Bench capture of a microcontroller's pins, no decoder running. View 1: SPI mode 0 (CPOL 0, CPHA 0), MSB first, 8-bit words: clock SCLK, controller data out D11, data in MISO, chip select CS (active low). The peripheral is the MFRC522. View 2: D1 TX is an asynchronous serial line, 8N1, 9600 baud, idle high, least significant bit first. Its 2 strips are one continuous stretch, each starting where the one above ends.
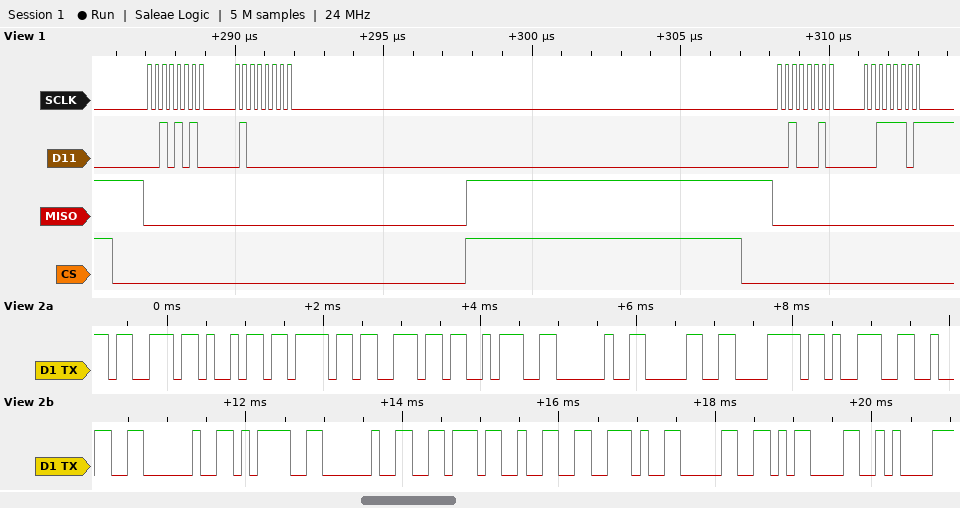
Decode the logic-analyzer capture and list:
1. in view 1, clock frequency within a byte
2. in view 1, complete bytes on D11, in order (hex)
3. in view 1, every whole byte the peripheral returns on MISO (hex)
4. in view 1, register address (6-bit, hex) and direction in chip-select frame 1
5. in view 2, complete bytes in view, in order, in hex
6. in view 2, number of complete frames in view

4 MHz
0x2A 0x40 0x22 0x3D
0x00 0x00 0x00 0x00
0x15 write
0x73 0x69 0x6F 0x6E 0x3A 0x20 0x30 0x78 0x39 0x32 0x20 0x3D 0x20 0x76 0x32 0x2E 0x30 0x0D 0x0A
19
